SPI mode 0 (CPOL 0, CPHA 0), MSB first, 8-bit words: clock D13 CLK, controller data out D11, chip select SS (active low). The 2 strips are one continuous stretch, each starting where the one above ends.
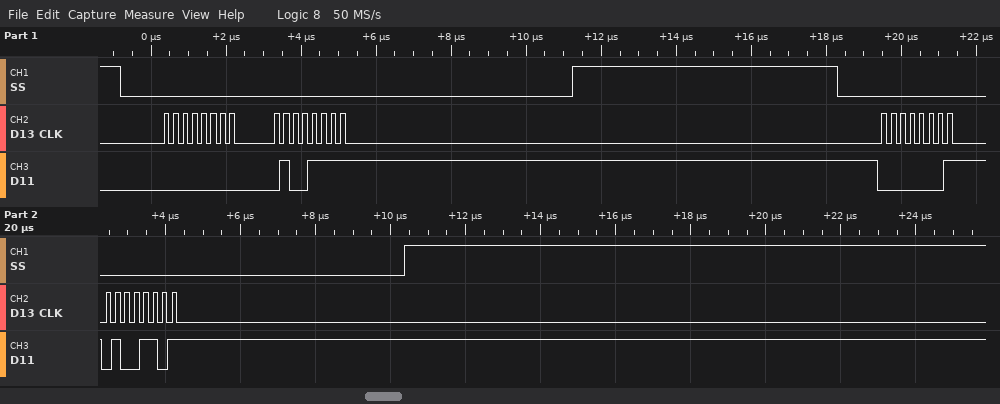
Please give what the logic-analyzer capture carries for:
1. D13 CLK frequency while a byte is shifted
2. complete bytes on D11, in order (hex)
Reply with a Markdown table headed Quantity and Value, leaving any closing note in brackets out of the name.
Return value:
| Quantity | Value |
|---|---|
| D13 CLK frequency while a byte is shifted | 4 MHz |
| complete bytes on D11, in order | 00 4F 01 4D |
